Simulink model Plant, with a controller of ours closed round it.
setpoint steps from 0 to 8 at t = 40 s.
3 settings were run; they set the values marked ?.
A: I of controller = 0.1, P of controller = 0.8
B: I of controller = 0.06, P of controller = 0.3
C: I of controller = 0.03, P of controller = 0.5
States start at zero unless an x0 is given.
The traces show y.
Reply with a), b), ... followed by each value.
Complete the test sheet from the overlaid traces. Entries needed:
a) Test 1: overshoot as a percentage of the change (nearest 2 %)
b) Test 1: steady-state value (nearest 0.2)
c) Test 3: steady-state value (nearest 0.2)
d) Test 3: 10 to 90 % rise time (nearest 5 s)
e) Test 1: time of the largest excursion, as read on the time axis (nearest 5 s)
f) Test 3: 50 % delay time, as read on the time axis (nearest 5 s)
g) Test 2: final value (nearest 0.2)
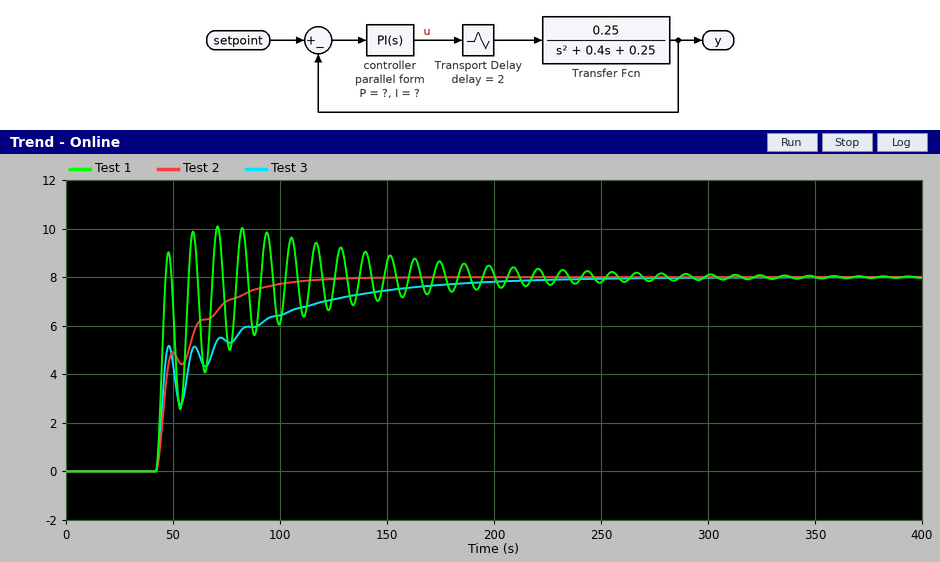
a) 26 %
b) 8.0
c) 8.0
d) 90 s
e) 70 s
f) 45 s
g) 8.0
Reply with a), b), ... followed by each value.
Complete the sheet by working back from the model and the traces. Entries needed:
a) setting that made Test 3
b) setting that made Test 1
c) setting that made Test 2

a) C
b) A
c) B
